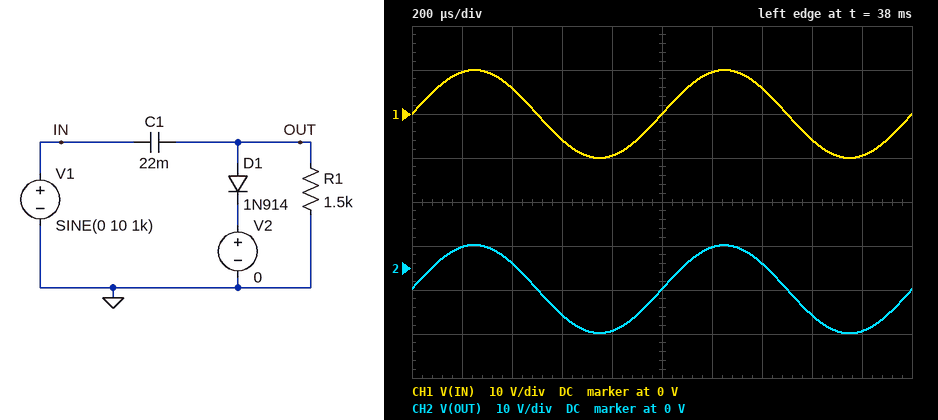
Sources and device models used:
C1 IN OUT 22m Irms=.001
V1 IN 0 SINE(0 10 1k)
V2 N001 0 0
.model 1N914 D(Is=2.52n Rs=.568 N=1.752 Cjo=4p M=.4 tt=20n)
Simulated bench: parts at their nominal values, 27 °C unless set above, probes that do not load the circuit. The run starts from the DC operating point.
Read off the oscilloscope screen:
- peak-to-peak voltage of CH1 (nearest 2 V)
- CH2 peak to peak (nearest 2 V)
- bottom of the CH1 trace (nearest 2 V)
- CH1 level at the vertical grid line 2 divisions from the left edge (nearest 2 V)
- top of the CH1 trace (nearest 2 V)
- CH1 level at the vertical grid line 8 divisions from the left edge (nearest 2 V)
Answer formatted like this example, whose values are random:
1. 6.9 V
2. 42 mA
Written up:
1. 20 V
2. 20 V
3. -10 V
4. 6 V
5. 10 V
6. -6 V
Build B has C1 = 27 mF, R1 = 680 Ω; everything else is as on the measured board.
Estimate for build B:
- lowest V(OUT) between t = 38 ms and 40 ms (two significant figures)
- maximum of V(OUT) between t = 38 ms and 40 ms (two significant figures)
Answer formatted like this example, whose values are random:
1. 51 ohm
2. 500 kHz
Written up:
1. -14 V
2. 5.8 V
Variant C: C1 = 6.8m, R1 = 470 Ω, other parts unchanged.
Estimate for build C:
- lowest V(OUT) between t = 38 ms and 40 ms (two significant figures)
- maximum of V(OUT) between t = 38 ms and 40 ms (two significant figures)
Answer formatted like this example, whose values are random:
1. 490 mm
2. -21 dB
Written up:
1. -18 V
2. 2.5 V
